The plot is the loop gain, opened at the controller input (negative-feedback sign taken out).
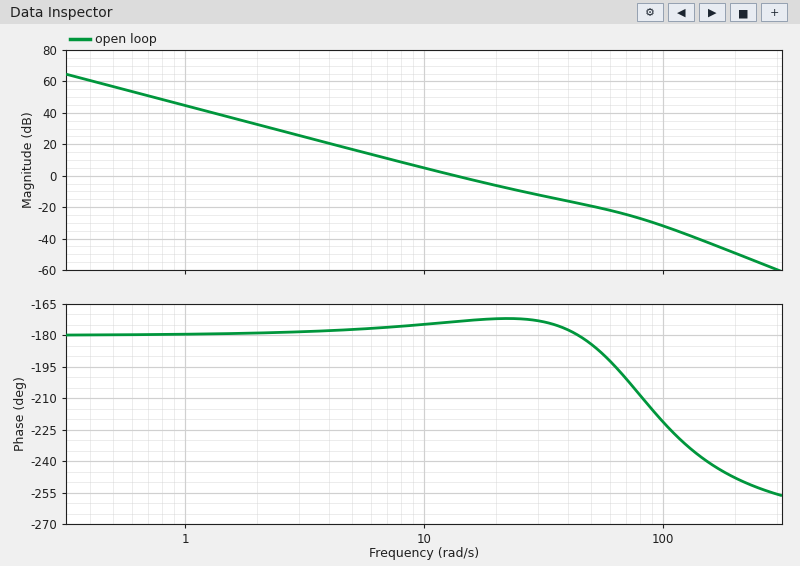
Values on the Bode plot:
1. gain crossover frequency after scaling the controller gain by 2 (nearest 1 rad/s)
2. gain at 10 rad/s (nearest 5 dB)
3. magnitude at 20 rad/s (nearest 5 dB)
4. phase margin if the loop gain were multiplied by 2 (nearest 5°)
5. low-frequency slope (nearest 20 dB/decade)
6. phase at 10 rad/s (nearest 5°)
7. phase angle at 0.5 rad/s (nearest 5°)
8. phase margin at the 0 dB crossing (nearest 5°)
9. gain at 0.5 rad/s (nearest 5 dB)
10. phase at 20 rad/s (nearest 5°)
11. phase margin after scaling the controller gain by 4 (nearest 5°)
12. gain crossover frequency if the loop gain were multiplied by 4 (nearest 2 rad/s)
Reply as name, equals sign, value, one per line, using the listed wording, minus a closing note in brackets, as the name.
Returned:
gain crossover frequency after scaling the controller gain by 2 = 20 rad/s
gain at 10 rad/s = 5 dB
magnitude at 20 rad/s = -5 dB
phase margin if the loop gain were multiplied by 2 = 10°
low-frequency slope = -40 dB/decade
phase at 10 rad/s = -175°
phase angle at 0.5 rad/s = -180°
phase margin at the 0 dB crossing = 5°
gain at 0.5 rad/s = 55 dB
phase at 20 rad/s = -170°
phase margin after scaling the controller gain by 4 = 5°
gain crossover frequency if the loop gain were multiplied by 4 = 30 rad/s
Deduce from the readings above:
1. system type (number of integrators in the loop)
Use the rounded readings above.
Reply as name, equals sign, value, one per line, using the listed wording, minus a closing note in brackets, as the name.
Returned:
system type = 2
